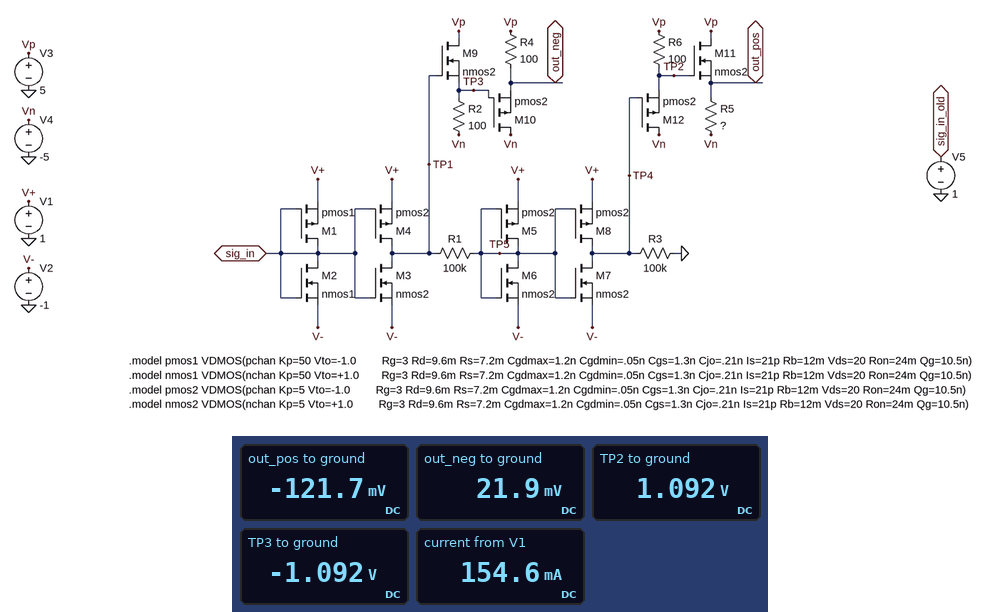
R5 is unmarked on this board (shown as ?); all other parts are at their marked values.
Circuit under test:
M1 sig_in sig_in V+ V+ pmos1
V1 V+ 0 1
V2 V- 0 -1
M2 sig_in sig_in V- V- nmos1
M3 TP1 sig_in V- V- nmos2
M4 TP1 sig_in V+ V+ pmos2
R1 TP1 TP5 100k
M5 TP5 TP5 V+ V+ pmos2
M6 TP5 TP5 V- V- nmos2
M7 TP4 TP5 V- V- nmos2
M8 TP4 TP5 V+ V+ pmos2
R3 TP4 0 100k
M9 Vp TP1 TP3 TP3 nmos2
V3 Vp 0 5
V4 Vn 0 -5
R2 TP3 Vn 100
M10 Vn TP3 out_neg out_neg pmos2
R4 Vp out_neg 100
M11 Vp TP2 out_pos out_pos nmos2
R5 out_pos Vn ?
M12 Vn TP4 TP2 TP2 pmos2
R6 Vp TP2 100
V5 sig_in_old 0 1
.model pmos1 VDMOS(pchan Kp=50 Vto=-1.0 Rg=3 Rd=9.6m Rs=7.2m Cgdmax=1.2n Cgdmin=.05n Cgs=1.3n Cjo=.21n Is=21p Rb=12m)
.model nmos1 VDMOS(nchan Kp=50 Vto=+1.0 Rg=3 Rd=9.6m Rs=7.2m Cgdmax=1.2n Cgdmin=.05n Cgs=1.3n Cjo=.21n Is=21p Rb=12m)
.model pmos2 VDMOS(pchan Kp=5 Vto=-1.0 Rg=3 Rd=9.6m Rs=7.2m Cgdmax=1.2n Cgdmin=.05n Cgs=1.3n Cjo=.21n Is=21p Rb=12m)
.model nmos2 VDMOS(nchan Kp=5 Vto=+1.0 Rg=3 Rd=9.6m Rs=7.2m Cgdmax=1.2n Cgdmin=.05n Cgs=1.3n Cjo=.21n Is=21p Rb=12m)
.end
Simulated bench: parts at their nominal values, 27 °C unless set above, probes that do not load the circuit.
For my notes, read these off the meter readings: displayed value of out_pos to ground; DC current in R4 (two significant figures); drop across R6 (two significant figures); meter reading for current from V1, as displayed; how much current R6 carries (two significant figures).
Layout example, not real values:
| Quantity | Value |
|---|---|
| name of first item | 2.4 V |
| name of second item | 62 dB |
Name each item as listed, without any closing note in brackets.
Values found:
| Quantity | Value |
|---|---|
| displayed value of out_pos to ground | -121.7 mV |
| DC current in R4 | 50 mA |
| drop across R6 | 3.9 V |
| meter reading for current from V1, as displayed | 154.6 mA |
| how much current R6 carries | 39 mA |
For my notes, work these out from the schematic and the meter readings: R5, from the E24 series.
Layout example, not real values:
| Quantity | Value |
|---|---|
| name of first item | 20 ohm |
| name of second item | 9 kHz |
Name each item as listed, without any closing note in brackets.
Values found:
| Quantity | Value |
|---|---|
| R5, from the E24 series | 39 Ω |
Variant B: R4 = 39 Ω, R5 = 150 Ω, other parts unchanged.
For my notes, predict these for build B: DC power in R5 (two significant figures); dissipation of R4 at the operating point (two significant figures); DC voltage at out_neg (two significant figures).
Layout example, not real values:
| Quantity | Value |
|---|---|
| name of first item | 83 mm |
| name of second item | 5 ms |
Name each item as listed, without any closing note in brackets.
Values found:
| Quantity | Value |
|---|---|
| DC power in R5 | 170 mW |
| dissipation of R4 at the operating point | 610 mW |
| DC voltage at out_neg | 120 mV |
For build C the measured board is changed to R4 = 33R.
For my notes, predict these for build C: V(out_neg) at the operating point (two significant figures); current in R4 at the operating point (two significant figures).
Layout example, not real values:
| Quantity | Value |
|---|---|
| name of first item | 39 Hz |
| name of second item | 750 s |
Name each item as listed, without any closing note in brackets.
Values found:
| Quantity | Value |
|---|---|
| V(out_neg) at the operating point | 140 mV |
| current in R4 at the operating point | 150 mA |
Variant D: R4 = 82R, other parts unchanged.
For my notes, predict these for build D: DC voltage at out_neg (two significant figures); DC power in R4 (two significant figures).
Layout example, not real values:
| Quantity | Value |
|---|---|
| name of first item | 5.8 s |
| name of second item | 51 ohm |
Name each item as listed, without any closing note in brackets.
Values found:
| Quantity | Value |
|---|---|
| DC voltage at out_neg | 41 mV |
| DC power in R4 | 300 mW |
